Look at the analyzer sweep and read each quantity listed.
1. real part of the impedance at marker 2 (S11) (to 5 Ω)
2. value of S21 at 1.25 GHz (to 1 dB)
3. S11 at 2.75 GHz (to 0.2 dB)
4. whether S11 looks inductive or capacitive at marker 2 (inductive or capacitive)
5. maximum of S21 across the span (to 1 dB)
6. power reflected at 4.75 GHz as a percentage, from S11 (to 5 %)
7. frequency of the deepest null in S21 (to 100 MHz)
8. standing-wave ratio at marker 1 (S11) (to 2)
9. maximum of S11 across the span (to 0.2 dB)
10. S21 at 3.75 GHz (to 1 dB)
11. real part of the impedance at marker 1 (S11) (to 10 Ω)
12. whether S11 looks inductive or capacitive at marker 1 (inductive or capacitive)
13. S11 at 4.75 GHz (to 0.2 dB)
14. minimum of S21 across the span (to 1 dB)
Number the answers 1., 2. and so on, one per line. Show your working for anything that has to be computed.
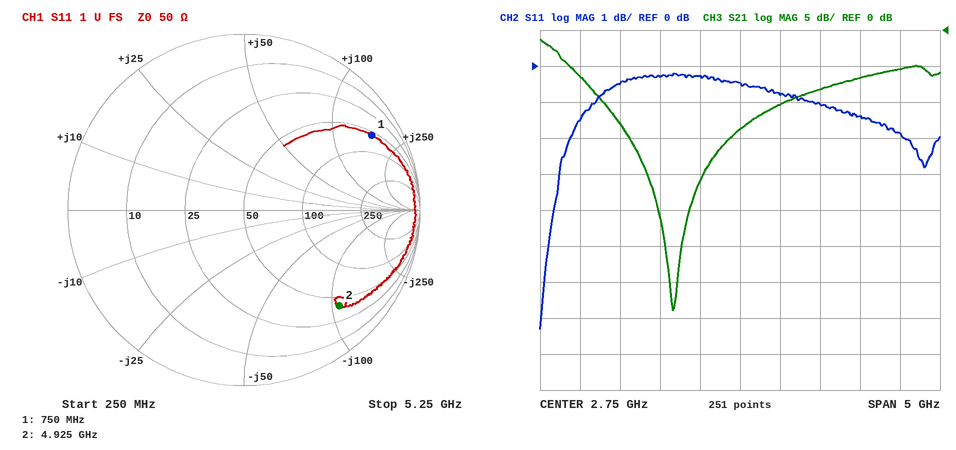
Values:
1. 40 Ω
2. -13 dB
3. -0.4 dB
4. capacitive
5. -1 dB
6. 10^(-1.8/10) ≈ 66.1 %, so 65 % to the nearest 5 %
7. 1.9 GHz
8. 12
9. -0.2 dB
10. -8 dB
11. 60 Ω
12. inductive
13. -1.8 dB
14. -39 dB
